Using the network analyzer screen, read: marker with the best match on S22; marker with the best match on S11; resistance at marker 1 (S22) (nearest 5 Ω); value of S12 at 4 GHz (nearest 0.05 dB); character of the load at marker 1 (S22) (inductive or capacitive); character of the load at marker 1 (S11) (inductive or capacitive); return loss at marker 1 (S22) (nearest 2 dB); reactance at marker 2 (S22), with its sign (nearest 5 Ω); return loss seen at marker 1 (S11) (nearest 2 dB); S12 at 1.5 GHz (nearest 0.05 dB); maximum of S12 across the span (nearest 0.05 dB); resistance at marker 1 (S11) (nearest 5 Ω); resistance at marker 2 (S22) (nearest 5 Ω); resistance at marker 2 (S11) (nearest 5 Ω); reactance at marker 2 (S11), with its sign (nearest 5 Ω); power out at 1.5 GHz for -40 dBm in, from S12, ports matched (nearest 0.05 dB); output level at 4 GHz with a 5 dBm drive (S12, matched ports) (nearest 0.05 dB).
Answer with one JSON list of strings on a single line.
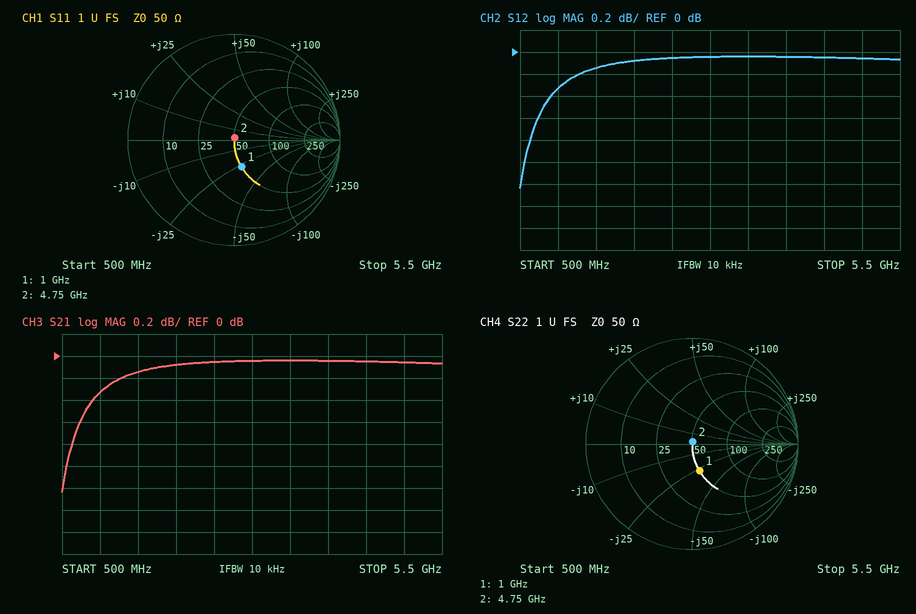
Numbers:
["marker 2", "marker 2", "50 Ω", "-0.05 dB", "capacitive", "capacitive", "12 dB", "0 Ω", "12 dB", "-0.15 dB", "-0.05 dB", "50 Ω", "50 Ω", "50 Ω", "0 Ω", "-40.15 dBm", "4.95 dBm"]
